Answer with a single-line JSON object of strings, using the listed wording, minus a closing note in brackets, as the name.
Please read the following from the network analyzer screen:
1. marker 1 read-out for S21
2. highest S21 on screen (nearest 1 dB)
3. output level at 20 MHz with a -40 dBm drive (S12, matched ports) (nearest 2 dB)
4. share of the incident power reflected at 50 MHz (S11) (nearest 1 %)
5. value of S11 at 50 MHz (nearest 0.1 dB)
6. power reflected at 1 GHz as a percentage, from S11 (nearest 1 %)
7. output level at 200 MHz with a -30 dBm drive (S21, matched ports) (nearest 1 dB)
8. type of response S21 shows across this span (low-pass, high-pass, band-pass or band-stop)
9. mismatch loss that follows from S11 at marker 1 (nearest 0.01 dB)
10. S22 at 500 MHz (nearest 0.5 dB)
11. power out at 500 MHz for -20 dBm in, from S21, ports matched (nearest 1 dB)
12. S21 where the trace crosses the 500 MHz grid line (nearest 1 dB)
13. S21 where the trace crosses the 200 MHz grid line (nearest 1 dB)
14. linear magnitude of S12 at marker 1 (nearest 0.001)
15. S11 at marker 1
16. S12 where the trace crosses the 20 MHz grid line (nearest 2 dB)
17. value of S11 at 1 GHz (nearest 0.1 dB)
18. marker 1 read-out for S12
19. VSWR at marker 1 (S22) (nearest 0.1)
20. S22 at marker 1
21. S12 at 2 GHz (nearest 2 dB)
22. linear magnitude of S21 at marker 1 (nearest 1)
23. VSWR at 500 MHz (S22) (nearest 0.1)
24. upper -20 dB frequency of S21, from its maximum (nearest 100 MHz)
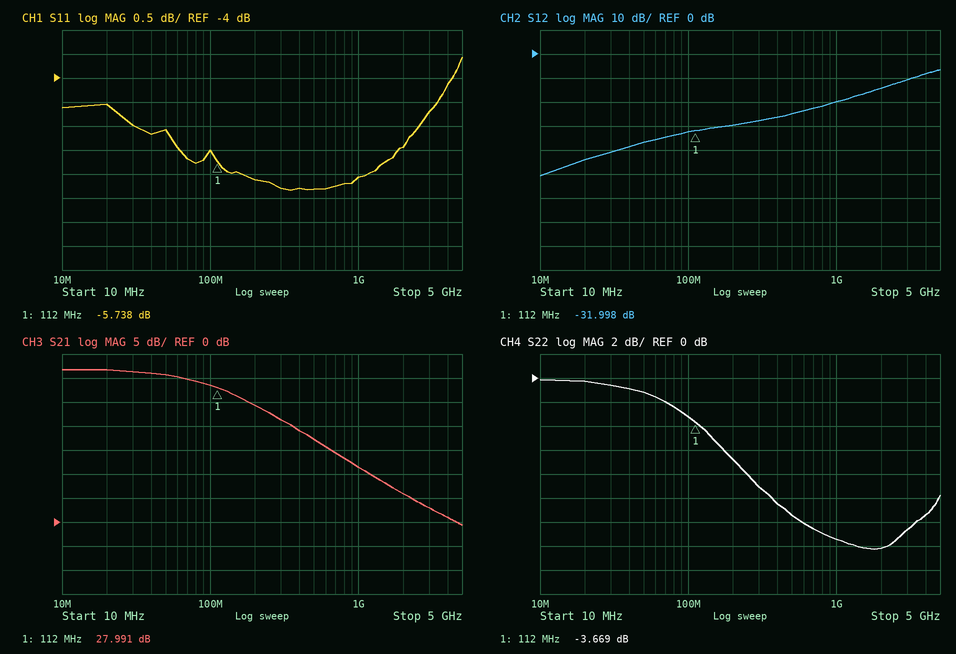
{"marker 1 read-out for S21": "27.991 dB", "highest S21 on screen": "32 dB", "output level at 20 MHz with a -40 dBm drive (S12, matched ports)": "-84 dBm", "share of the incident power reflected at 50 MHz (S11)": "31 %", "value of S11 at 50 MHz": "-5.1 dB", "power reflected at 1 GHz as a percentage, from S11": "25 %", "output level at 200 MHz with a -30 dBm drive (S21, matched ports)": "-6 dBm", "type of response S21 shows across this span": "low-pass", "mismatch loss that follows from S11 at marker 1": "1.35 dB", "S22 at 500 MHz": "-11.5 dB", "power out at 500 MHz for -20 dBm in, from S21, ports matched": "-3 dBm", "S21 where the trace crosses the 500 MHz grid line": "17 dB", "S21 where the trace crosses the 200 MHz grid line": "24 dB", "linear magnitude of S12 at marker 1": "0.025", "S11 at marker 1": "-5.738 dB", "S12 where the trace crosses the 20 MHz grid line": "-44 dB", "value of S11 at 1 GHz": "-6.1 dB", "marker 1 read-out for S12": "-31.998 dB", "VSWR at marker 1 (S22)": "4.8", "S22 at marker 1": "-3.669 dB", "S12 at 2 GHz": "-14 dB", "linear magnitude of S21 at marker 1": "25", "VSWR at 500 MHz (S22)": "1.7", "upper -20 dB frequency of S21, from its maximum": "1.0 GHz"}
